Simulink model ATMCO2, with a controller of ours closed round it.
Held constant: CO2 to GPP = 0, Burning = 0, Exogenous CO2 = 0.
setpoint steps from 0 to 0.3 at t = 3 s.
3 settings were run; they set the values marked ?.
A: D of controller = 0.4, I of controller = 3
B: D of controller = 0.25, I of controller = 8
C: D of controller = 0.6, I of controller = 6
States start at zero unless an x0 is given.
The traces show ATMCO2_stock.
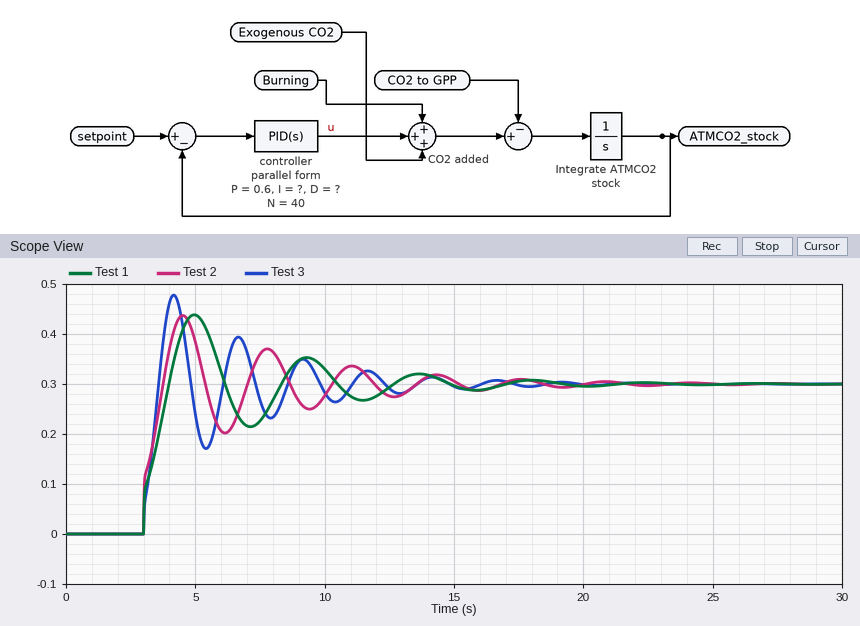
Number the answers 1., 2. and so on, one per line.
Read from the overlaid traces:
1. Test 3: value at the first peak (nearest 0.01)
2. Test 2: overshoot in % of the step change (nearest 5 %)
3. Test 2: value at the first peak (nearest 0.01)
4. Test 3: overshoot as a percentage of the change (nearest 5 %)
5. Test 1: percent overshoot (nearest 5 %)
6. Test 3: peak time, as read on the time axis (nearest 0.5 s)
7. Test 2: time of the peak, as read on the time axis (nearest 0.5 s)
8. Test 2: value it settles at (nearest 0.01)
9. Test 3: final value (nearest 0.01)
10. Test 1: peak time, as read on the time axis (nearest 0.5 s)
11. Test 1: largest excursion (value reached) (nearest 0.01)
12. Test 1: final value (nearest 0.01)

1. 0.48
2. 45 %
3. 0.44
4. 60 %
5. 45 %
6. 4.0 s
7. 4.5 s
8. 0.30
9. 0.30
10. 5.0 s
11. 0.44
12. 0.30
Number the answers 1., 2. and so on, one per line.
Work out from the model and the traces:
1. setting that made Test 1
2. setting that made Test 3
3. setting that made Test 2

1. A
2. B
3. C
